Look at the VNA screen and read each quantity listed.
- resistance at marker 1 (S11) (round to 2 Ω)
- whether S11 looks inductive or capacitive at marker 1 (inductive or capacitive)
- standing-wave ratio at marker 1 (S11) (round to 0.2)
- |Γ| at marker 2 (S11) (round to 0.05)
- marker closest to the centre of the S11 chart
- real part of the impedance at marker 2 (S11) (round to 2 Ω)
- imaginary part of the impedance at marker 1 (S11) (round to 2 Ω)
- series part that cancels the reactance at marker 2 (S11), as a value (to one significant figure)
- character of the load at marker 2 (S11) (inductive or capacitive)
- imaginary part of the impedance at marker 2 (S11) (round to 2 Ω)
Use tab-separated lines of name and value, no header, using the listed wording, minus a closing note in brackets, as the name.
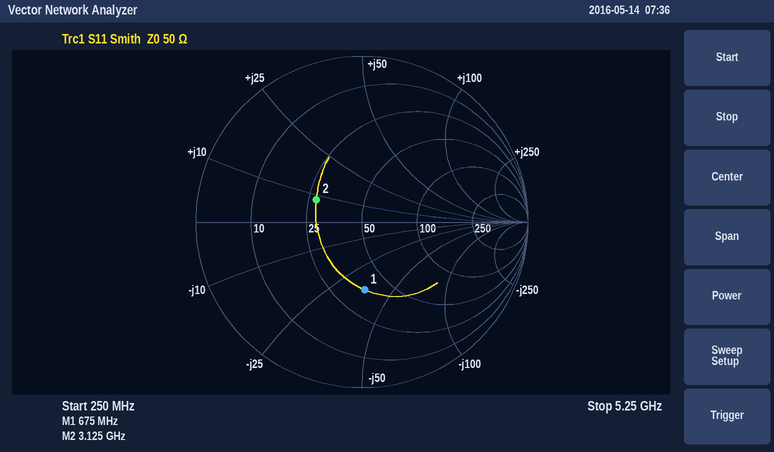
resistance at marker 1 (S11)	36 Ω
whether S11 looks inductive or capacitive at marker 1	capacitive
standing-wave ratio at marker 1 (S11)	2.4
|Γ| at marker 2 (S11)	0.30
marker closest to the centre of the S11 chart	marker 2
real part of the impedance at marker 2 (S11)	28 Ω
imaginary part of the impedance at marker 1 (S11)	-36 Ω
series part that cancels the reactance at marker 2 (S11), as a value	6 pF
character of the load at marker 2 (S11)	inductive
imaginary part of the impedance at marker 2 (S11)	+8 Ω
